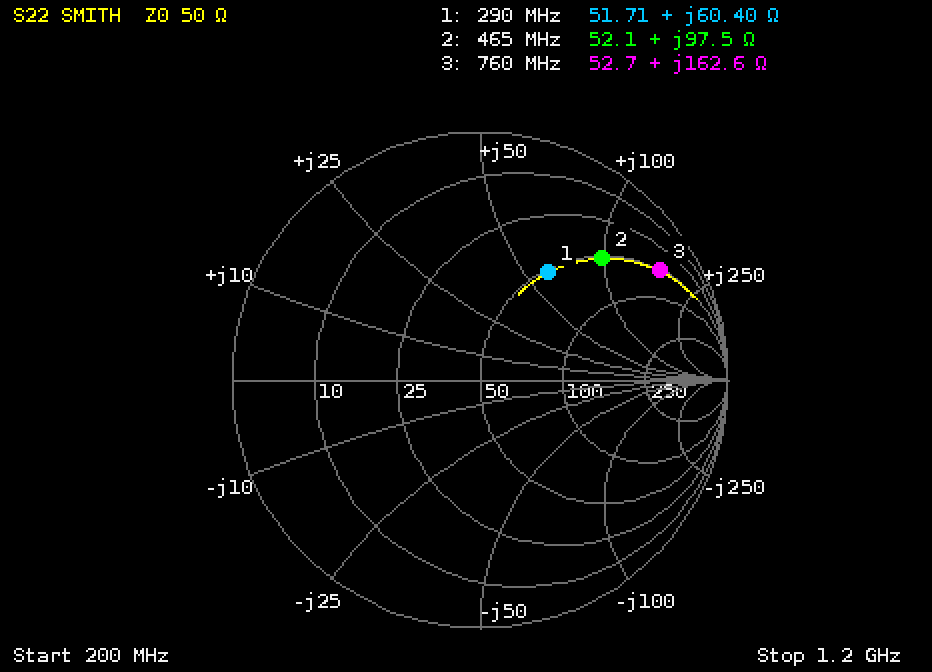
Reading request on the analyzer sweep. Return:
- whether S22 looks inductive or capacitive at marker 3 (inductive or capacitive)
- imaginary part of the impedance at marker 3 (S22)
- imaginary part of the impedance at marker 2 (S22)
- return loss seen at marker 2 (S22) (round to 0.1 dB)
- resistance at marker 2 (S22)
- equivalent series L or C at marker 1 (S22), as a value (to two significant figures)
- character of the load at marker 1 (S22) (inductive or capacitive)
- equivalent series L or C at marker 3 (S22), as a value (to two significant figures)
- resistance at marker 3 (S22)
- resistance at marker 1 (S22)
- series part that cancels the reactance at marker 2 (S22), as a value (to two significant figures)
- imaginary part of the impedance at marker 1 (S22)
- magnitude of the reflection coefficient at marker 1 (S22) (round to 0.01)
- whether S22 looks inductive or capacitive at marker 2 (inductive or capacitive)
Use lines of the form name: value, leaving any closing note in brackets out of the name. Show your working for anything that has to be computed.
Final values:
whether S22 looks inductive or capacitive at marker 3: inductive
imaginary part of the impedance at marker 3: +162.6 Ω
imaginary part of the impedance at marker 2: +97.5 Ω
return loss seen at marker 2 (S22): 3.2 dB
resistance at marker 2: 52.1 Ω
equivalent series L or C at marker 1 (S22), as a value: L = 60.4 Ω/(2π × 290 MHz) ≈ 33 nH
character of the load at marker 1 (S22): inductive
equivalent series L or C at marker 3 (S22), as a value: L = 162.6 Ω/(2π × 760 MHz) ≈ 34 nH
resistance at marker 3: 52.7 Ω
resistance at marker 1: 51.71 Ω
series part that cancels the reactance at marker 2 (S22), as a value: C = 1/(2π × 465 MHz × 97.5 Ω) ≈ 3.5 pF
imaginary part of the impedance at marker 1: +60.40 Ω
magnitude of the reflection coefficient at marker 1 (S22): 0.51
whether S22 looks inductive or capacitive at marker 2: inductive
